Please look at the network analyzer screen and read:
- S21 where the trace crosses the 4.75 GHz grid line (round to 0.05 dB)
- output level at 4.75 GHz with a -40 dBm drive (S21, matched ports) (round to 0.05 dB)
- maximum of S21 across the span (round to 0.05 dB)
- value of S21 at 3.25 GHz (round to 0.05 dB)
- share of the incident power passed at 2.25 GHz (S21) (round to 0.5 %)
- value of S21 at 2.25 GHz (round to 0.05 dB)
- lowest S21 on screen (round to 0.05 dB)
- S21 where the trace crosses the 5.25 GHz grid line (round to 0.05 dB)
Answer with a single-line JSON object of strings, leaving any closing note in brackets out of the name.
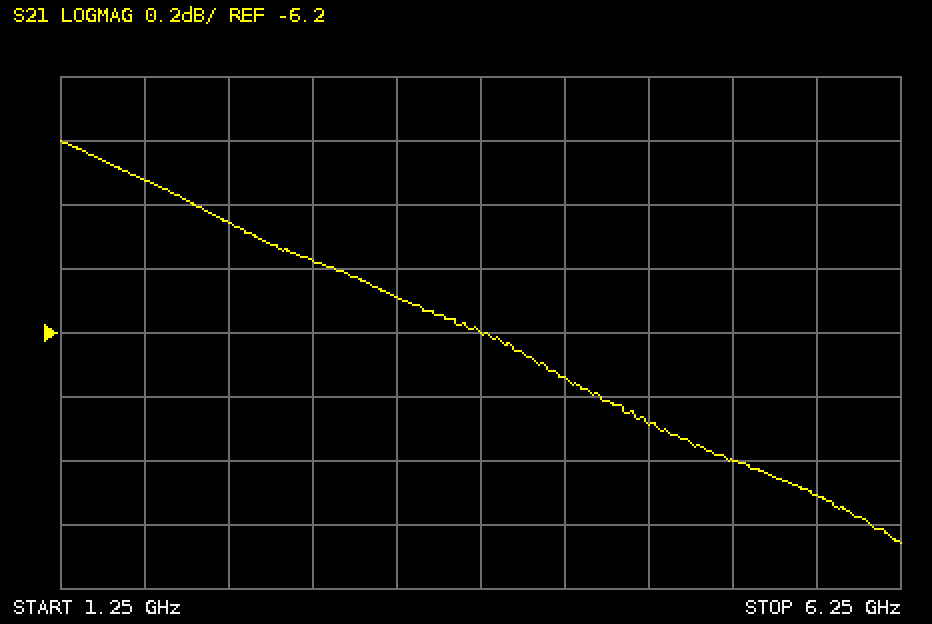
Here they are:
{"S21 where the trace crosses the 4.75 GHz grid line": "-6.50 dB", "output level at 4.75 GHz with a -40 dBm drive (S21, matched ports)": "-46.50 dBm", "maximum of S21 across the span": "-5.60 dB", "value of S21 at 3.25 GHz": "-6.10 dB", "share of the incident power passed at 2.25 GHz (S21)": "26.0 %", "value of S21 at 2.25 GHz": "-5.85 dB", "lowest S21 on screen": "-6.85 dB", "S21 where the trace crosses the 5.25 GHz grid line": "-6.60 dB"}
